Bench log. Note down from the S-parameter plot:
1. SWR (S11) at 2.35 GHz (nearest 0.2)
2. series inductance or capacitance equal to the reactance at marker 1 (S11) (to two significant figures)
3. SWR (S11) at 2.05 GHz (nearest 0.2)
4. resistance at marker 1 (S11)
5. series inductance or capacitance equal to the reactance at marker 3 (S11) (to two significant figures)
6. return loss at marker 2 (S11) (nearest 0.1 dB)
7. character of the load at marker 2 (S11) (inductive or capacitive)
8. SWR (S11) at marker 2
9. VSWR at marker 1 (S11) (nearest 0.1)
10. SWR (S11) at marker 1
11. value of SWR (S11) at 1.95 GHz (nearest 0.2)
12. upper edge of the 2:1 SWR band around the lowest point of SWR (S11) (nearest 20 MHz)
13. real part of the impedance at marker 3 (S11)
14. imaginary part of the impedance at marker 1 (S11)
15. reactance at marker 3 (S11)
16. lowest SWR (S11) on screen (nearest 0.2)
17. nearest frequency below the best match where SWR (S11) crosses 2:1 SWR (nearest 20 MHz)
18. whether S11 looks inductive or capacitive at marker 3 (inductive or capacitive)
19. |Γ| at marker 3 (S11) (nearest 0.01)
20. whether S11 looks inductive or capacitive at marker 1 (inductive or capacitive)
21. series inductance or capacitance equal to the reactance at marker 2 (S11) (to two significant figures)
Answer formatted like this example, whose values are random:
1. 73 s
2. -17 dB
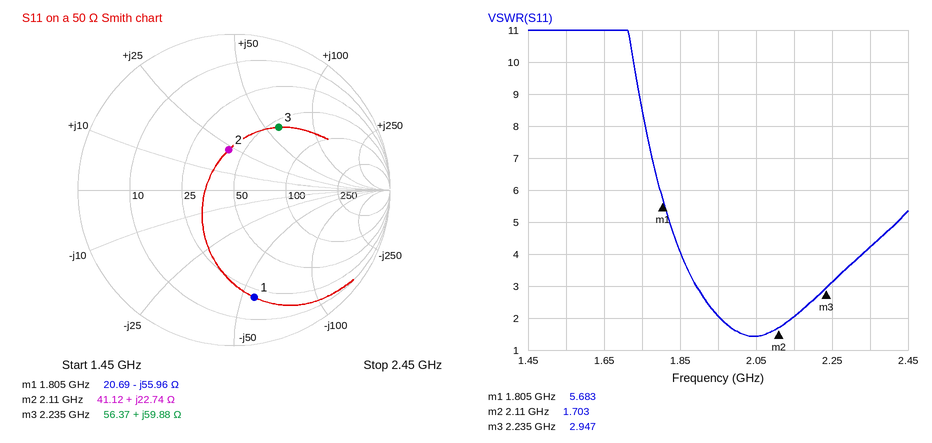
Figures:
1. 4.2
2. 1.6 pF
3. 1.4
4. 20.69 Ω
5. 4.3 nH
6. 11.7 dB
7. inductive
8. 1.703
9. 5.7
10. 5.683
11. 2.0
12. 2.14 GHz
13. 56.37 Ω
14. -55.96 Ω
15. +59.88 Ω
16. 1.4
17. 1.96 GHz
18. inductive
19. 0.49
20. capacitive
21. 1.7 nH
